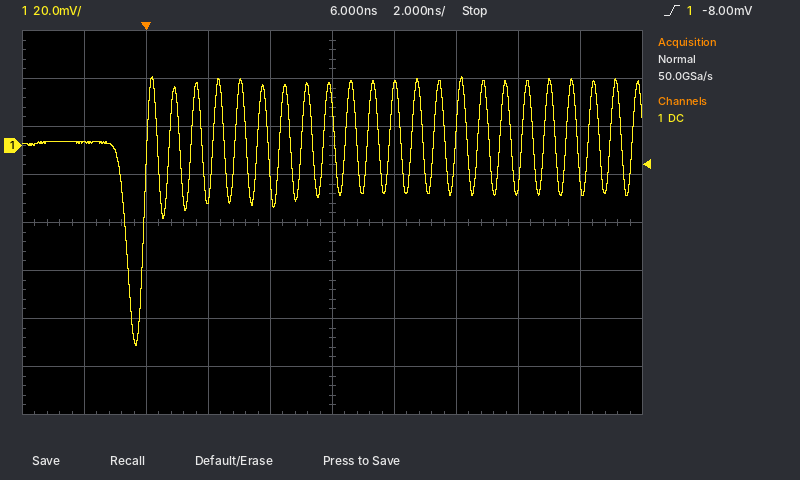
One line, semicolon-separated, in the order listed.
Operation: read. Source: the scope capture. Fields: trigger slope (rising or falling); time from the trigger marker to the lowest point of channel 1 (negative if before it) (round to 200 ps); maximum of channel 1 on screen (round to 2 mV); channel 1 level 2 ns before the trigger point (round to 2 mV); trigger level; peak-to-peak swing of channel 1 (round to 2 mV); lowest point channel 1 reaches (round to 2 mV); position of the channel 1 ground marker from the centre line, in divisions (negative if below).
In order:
rising; -400 ps; 28 mV; 2 mV; -8.00 mV; 112 mV; -84 mV; +1.6 div
